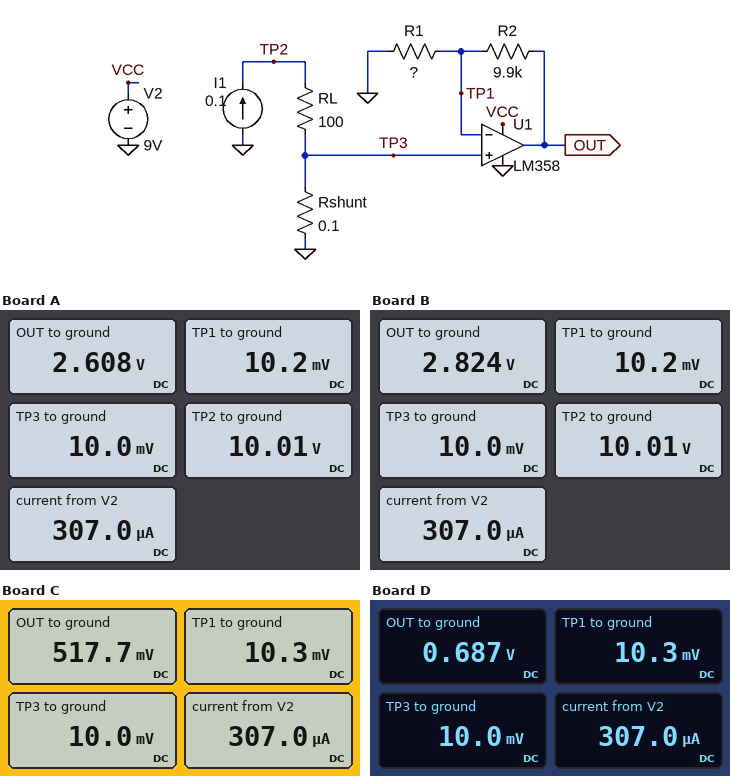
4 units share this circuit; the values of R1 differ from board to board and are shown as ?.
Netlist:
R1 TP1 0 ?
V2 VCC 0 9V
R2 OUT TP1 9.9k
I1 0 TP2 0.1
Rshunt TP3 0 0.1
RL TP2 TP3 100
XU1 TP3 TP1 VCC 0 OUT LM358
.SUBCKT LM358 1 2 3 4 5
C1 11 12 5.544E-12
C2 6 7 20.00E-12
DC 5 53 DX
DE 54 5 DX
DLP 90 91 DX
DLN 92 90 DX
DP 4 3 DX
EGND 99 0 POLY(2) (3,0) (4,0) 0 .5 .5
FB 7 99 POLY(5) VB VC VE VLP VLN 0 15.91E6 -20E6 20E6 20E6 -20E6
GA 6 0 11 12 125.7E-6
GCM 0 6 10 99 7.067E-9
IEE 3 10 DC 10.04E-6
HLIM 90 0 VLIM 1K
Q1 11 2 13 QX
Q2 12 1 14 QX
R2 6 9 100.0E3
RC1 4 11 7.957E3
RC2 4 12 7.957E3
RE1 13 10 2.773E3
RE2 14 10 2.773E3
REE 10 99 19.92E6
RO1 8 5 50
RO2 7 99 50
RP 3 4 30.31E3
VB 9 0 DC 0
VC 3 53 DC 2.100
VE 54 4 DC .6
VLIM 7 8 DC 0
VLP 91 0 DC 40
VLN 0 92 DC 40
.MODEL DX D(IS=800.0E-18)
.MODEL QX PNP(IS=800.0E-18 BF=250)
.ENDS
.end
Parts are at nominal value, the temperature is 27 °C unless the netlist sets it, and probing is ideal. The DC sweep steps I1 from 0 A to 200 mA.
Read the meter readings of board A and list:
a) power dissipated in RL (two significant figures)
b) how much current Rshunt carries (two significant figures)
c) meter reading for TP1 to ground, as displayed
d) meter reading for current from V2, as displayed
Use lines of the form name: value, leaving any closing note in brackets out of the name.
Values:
power dissipated in RL: 1.0 W
how much current Rshunt carries: 100 mA
meter reading for TP1 to ground, as displayed: 10.2 mV
meter reading for current from V2, as displayed: 307.0 µA
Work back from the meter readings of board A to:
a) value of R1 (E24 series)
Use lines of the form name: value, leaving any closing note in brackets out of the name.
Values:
value of R1: 39 Ω
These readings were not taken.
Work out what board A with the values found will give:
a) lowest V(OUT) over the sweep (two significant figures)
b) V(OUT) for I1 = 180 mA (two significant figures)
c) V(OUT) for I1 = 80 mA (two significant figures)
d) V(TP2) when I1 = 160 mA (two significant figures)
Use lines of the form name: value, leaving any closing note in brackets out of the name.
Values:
lowest V(OUT) over the sweep: 150 mV
V(OUT) for I1 = 180 mA: 4.6 V
V(OUT) for I1 = 80 mA: 2.1 V
V(TP2) when I1 = 160 mA: 16 V
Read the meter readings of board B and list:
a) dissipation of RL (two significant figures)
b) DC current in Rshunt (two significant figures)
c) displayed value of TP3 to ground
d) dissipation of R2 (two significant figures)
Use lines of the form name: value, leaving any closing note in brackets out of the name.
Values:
dissipation of RL: 1.0 W
DC current in Rshunt: 100 mA
displayed value of TP3 to ground: 10.0 mV
dissipation of R2: 800 µW
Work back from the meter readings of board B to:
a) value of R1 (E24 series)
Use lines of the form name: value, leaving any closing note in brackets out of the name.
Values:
value of R1: 36 Ω
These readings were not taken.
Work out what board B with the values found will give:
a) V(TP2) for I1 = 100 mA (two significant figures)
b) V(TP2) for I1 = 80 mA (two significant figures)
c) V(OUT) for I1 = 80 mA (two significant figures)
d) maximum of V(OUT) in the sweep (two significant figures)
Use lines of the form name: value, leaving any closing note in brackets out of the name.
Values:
V(TP2) for I1 = 100 mA: 10 V
V(TP2) for I1 = 80 mA: 8.0 V
V(OUT) for I1 = 80 mA: 2.3 V
maximum of V(OUT) in the sweep: 5.6 V
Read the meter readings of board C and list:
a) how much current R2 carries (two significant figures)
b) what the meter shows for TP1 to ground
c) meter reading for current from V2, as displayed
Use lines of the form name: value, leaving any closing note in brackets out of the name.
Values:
how much current R2 carries: 51 µA
what the meter shows for TP1 to ground: 10.3 mV
meter reading for current from V2, as displayed: 307.0 µA
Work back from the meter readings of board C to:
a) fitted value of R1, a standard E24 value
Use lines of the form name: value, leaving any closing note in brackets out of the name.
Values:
fitted value of R1, a standard E24 value: 200 Ω
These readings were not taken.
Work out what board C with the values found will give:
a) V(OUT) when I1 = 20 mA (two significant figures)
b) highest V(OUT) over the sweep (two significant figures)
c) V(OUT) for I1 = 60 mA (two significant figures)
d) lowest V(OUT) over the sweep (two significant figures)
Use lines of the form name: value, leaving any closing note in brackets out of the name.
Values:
V(OUT) when I1 = 20 mA: 140 mV
highest V(OUT) over the sweep: 1.0 V
V(OUT) for I1 = 60 mA: 320 mV
lowest V(OUT) over the sweep: 100 mV
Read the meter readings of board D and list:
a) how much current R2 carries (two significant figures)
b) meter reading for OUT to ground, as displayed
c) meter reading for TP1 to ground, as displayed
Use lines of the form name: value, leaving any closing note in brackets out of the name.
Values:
how much current R2 carries: 68 µA
meter reading for OUT to ground, as displayed: 0.687 V
meter reading for TP1 to ground, as displayed: 10.3 mV
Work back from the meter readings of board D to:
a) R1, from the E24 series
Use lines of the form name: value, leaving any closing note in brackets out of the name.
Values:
R1, from the E24 series: 150 Ω
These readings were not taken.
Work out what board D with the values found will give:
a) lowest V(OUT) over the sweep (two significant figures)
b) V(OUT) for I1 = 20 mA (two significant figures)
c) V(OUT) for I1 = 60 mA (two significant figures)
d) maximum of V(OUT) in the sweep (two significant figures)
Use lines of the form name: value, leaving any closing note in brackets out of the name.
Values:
lowest V(OUT) over the sweep: 110 mV
V(OUT) for I1 = 20 mA: 160 mV
V(OUT) for I1 = 60 mA: 420 mV
maximum of V(OUT) in the sweep: 1.4 V
